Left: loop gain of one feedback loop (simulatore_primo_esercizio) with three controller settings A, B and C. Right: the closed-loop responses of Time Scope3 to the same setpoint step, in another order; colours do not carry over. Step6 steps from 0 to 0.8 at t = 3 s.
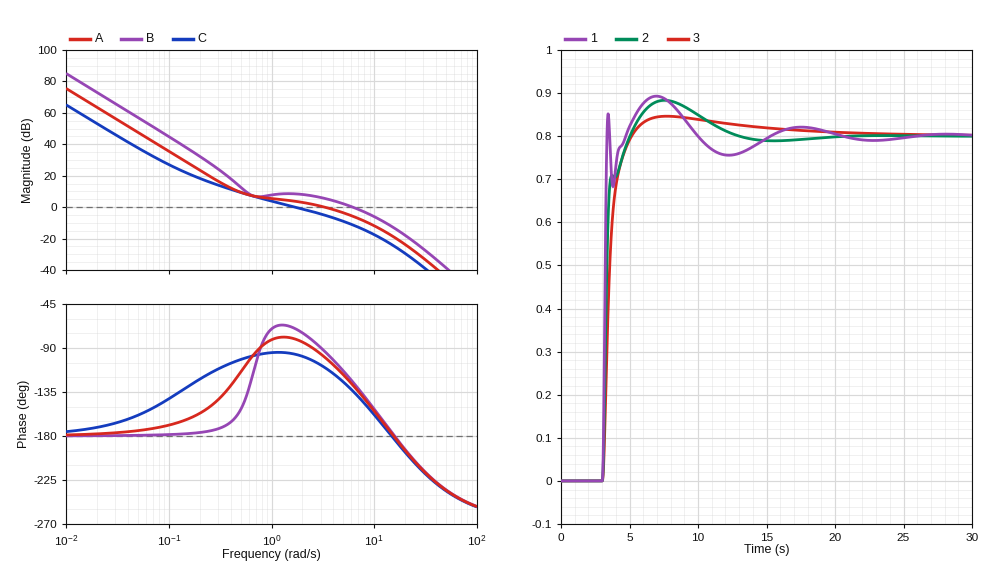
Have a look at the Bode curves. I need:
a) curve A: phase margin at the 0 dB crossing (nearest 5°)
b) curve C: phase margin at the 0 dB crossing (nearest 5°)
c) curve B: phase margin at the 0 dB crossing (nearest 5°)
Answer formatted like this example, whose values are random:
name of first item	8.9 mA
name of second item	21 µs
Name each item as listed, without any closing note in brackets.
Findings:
curve A: phase margin at the 0 dB crossing	80°
curve C: phase margin at the 0 dB crossing	85°
curve B: phase margin at the 0 dB crossing	55°
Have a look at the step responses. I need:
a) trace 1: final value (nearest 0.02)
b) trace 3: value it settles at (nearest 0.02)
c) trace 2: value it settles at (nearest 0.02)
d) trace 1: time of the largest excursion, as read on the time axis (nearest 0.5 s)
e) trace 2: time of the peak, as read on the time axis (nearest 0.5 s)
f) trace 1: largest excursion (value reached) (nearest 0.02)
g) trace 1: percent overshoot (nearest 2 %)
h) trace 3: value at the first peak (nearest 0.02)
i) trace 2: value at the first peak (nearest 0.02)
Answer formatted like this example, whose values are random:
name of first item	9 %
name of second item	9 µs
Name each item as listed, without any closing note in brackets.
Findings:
trace 1: final value	0.80
trace 3: value it settles at	0.80
trace 2: value it settles at	0.80
trace 1: time of the largest excursion, as read on the time axis	7.0 s
trace 2: time of the peak, as read on the time axis	7.5 s
trace 1: largest excursion (value reached)	0.90
trace 1: percent overshoot	12 %
trace 3: value at the first peak	0.84
trace 2: value at the first peak	0.88
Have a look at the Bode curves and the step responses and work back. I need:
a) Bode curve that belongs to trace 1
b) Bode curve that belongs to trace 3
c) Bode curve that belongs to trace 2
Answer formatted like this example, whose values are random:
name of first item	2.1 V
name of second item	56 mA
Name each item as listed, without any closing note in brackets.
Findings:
Bode curve that belongs to trace 1	B
Bode curve that belongs to trace 3	C
Bode curve that belongs to trace 2	A
